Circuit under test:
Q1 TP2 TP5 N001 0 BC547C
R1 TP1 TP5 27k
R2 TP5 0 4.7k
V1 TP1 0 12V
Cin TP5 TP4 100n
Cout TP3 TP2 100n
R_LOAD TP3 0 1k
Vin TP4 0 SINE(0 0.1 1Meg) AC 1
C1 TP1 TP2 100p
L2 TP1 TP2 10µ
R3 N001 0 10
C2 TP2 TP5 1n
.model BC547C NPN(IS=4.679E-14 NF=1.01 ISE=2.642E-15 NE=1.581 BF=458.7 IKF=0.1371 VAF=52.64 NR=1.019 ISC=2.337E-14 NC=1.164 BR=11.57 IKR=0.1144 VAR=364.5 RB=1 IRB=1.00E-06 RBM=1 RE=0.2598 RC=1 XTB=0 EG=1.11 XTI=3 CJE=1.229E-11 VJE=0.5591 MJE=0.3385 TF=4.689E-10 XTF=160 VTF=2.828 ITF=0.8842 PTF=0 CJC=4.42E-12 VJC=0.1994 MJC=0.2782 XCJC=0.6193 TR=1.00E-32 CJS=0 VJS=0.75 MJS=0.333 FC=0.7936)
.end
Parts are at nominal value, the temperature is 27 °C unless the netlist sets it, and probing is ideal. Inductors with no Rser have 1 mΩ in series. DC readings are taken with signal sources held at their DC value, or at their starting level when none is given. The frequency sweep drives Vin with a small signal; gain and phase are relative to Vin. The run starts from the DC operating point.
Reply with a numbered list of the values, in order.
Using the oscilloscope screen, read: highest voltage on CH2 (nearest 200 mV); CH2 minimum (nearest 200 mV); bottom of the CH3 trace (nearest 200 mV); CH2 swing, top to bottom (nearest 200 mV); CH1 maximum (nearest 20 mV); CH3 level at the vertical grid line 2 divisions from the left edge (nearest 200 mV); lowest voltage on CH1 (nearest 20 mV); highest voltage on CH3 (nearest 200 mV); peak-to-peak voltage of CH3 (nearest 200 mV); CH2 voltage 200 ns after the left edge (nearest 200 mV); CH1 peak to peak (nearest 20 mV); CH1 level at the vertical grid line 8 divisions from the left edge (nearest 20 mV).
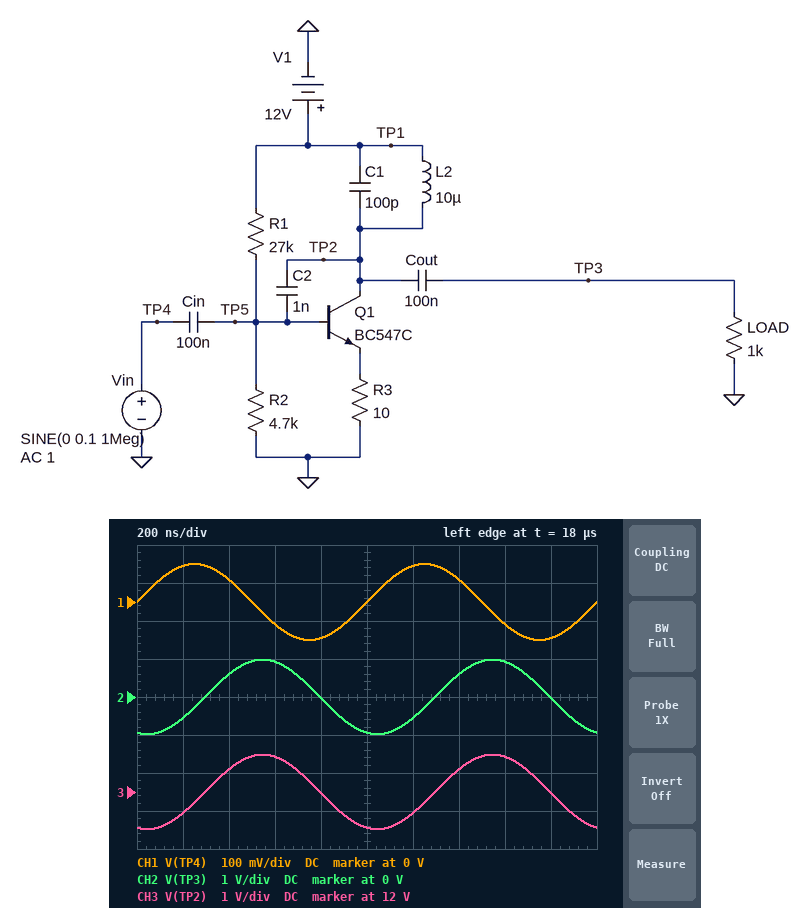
1. 1.0 V
2. -1.0 V
3. 11.0 V
4. 2.0 V
5. 100 mV
6. 12.6 V
7. -100 mV
8. 13.0 V
9. 2.0 V
10. -600 mV
11. 200 mV
12. -60 mV
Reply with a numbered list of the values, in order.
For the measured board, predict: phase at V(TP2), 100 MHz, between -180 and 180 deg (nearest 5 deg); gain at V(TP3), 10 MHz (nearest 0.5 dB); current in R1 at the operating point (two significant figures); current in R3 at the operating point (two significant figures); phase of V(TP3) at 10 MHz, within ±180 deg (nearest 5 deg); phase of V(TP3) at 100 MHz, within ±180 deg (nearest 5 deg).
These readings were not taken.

1. 5 deg
2. 4.5 dB
3. 400 µA
4. 53 mA
5. 55 deg
6. 5 deg
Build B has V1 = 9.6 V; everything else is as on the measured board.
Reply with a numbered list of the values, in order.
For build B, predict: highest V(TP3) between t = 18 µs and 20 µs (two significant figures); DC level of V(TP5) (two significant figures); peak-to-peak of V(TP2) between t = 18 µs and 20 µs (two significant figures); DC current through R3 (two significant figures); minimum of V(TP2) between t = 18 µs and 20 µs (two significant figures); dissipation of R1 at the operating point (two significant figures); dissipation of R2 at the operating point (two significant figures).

1. 960 mV
2. 1.1 V
3. 1.9 V
4. 36 mA
5. 8.6 V
6. 2.7 mW
7. 250 µW
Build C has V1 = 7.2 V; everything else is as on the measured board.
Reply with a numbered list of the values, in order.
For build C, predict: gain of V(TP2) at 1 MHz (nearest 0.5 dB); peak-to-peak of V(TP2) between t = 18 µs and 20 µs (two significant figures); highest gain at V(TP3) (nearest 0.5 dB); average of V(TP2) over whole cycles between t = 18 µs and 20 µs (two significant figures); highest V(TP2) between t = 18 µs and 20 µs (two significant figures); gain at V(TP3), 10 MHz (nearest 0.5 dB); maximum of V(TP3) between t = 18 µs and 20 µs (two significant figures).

1. 19.0 dB
2. 1.8 V
3. 33.0 dB
4. 7.2 V
5. 8.1 V
6. 4.0 dB
7. 920 mV
